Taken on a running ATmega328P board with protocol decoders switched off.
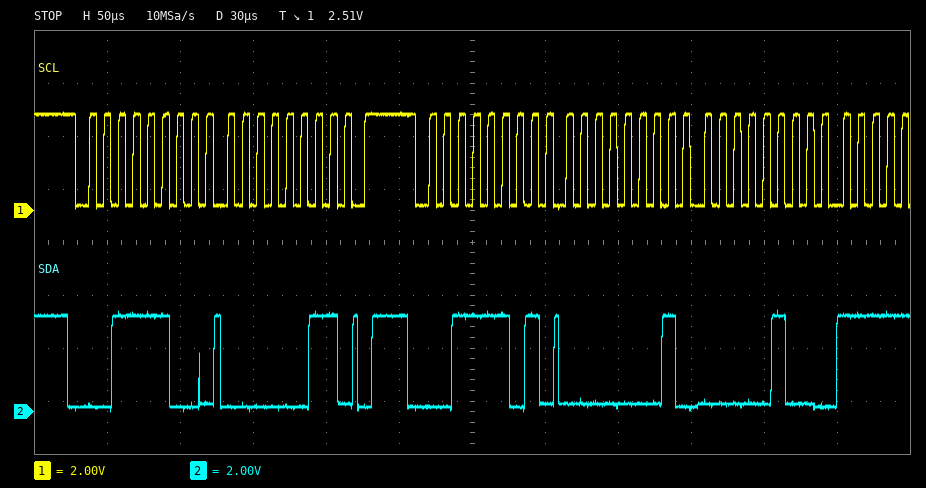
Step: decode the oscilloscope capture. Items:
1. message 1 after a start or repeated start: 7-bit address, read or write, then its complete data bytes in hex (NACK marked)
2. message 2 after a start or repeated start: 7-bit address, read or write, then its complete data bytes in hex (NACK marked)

0x1E write: 03
0x1E read: 01 04
